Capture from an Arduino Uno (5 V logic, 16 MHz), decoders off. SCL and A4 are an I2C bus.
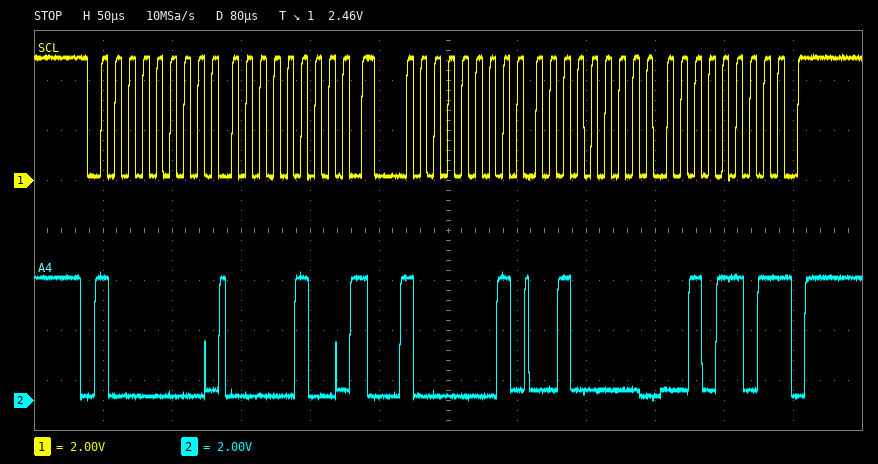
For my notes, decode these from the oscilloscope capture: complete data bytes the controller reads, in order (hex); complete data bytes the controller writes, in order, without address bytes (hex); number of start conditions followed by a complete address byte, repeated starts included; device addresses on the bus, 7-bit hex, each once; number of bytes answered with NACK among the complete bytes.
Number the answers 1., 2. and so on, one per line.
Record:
1. 20 2D
2. 04
3. 2
4. 0x40
5. 1
